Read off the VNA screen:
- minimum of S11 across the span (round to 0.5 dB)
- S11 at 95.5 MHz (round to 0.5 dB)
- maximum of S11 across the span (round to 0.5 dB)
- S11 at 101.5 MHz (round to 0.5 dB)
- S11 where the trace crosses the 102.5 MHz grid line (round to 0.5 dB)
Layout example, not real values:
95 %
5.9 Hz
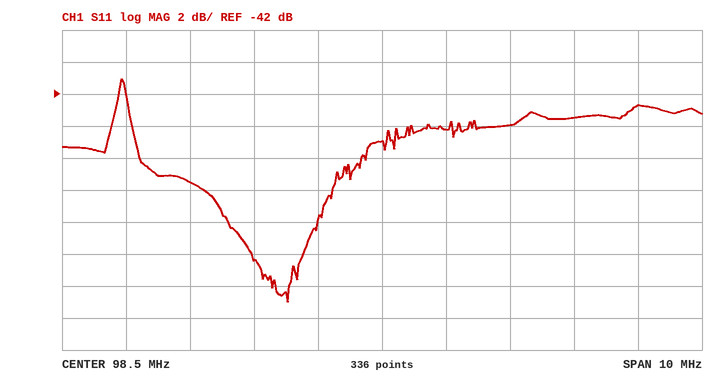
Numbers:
-55.0 dB
-47.5 dB
-41.0 dB
-43.5 dB
-42.5 dB
